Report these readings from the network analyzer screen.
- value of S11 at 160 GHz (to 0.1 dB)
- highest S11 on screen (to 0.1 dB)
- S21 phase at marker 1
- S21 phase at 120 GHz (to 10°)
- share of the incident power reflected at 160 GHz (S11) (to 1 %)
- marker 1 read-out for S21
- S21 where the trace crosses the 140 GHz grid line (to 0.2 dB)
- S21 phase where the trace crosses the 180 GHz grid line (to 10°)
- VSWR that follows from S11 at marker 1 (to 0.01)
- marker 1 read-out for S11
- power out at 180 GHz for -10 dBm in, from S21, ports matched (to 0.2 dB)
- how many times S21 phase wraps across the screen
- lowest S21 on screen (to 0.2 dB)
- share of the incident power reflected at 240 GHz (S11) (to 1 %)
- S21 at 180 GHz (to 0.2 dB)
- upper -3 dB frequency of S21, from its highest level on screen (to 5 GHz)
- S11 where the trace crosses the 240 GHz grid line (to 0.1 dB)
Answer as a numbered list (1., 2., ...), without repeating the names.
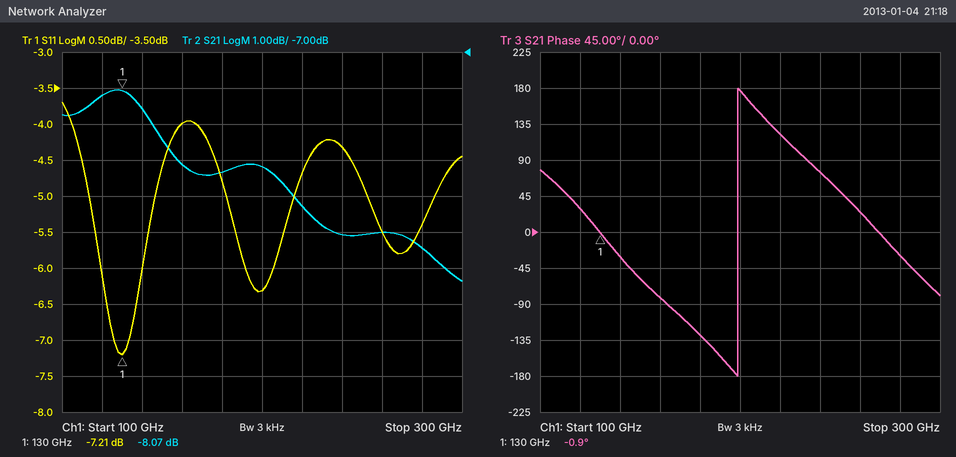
1. -4.0 dB
2. -3.7 dB
3. -0.9°
4. 30°
5. 40 %
6. -8.07 dB
7. -8.6 dB
8. -130°
9. 2.55
10. -7.21 dB
11. -20.4 dBm
12. 1
13. -13.4 dB
14. 37 %
15. -10.4 dB
16. 215 GHz
17. -4.3 dB
